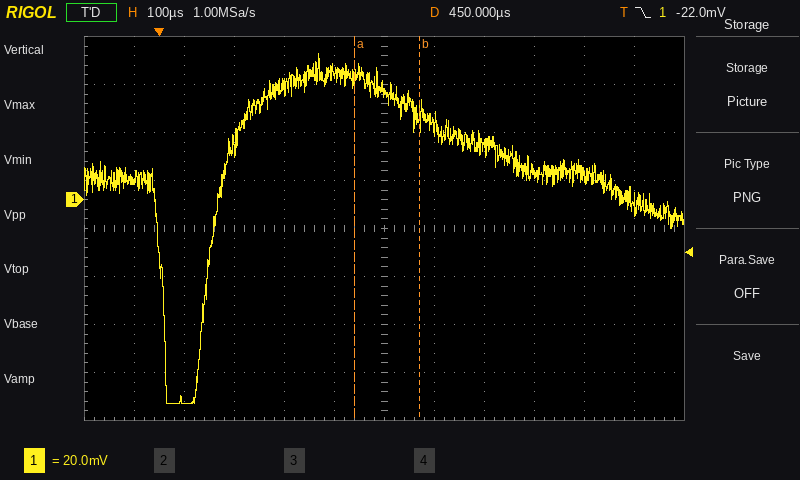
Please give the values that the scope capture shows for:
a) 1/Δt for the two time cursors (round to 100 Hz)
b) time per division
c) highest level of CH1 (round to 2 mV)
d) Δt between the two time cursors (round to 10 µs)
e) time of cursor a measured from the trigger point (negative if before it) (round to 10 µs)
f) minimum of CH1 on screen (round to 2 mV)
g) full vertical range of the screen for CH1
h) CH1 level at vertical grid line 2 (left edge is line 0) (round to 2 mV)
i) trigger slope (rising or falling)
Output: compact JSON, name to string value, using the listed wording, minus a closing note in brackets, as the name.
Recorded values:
{"1/Δt for the two time cursors": "7.7 kHz", "time per division": "100 µs", "highest level of CH1": "60 mV", "Δt between the two time cursors": "130 µs", "time of cursor a measured from the trigger point (negative if before it)": "+390 µs", "minimum of CH1 on screen": "-84 mV", "full vertical range of the screen for CH1": "160 mV", "CH1 level at vertical grid line 2 (left edge is line 0)": "-84 mV", "trigger slope": "falling"}
